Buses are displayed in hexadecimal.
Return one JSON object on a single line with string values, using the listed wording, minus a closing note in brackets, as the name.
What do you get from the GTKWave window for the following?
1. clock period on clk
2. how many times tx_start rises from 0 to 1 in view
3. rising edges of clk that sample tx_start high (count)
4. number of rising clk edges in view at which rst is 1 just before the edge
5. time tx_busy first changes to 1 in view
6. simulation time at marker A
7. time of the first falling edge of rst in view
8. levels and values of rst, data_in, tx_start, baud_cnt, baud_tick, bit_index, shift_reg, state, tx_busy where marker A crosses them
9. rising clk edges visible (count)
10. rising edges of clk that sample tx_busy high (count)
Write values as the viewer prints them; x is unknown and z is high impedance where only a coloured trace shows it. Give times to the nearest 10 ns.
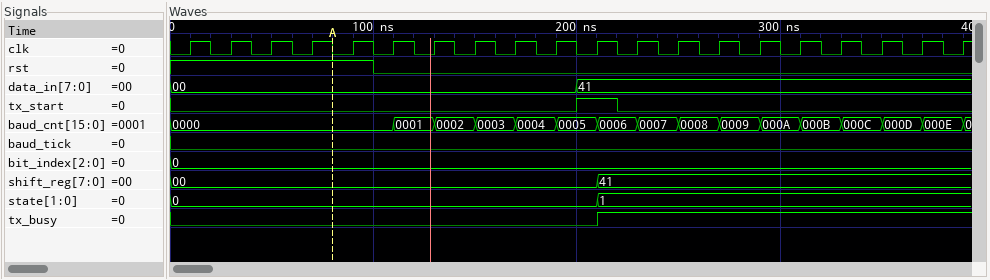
{"clock period on clk": "20 ns", "how many times tx_start rises from 0 to 1 in view": "1", "rising edges of clk that sample tx_start high": "1", "number of rising clk edges in view at which rst is 1 just before the edge": "5", "time tx_busy first changes to 1 in view": "210 ns", "simulation time at marker A": "80 ns", "time of the first falling edge of rst in view": "100 ns", "levels and values of rst, data_in, tx_start, baud_cnt, baud_tick, bit_index, shift_reg, state, tx_busy where marker A crosses them": "rst=1, data_in=00, tx_start=0, baud_cnt=0000, baud_tick=0, bit_index=0, shift_reg=00, state=0, tx_busy=0", "rising clk edges visible": "20", "rising edges of clk that sample tx_busy high": "9"}
